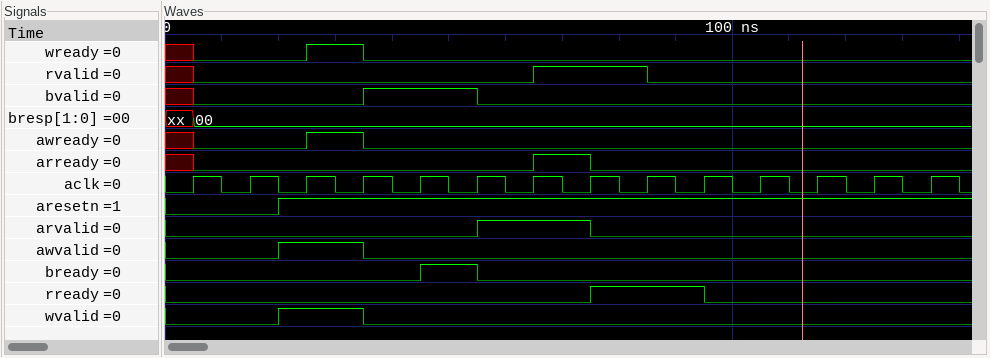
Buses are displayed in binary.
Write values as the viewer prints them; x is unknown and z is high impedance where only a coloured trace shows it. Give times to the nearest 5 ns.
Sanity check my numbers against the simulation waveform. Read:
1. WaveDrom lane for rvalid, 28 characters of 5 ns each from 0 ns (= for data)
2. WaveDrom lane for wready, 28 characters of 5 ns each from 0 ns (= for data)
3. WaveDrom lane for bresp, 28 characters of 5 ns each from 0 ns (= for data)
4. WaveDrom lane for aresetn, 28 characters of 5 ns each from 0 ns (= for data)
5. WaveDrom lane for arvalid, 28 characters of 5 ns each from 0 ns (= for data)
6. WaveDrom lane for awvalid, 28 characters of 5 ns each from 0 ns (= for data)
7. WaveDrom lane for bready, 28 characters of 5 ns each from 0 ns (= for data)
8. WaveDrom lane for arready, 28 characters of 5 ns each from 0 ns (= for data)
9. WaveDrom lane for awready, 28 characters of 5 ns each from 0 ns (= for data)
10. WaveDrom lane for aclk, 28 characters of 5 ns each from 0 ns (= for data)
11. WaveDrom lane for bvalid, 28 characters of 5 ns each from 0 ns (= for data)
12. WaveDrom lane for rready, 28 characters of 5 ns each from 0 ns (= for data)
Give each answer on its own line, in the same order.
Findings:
{name: 'rvalid', wave: 'x0...........1...0..........'}
{name: 'wready', wave: 'x0...1.0....................'}
{name: 'bresp', wave: 'x=..........................', data: '00'}
{name: 'aresetn', wave: '0...1.......................'}
{name: 'arvalid', wave: '0..........1...0............'}
{name: 'awvalid', wave: '0...1..0....................'}
{name: 'bready', wave: '0........1.0................'}
{name: 'arready', wave: 'x0...........1.0............'}
{name: 'awready', wave: 'x0...1.0....................'}
{name: 'aclk', wave: '0101010101010101010101010101'}
{name: 'bvalid', wave: 'x0.....1...0................'}
{name: 'rready', wave: '0..............1...0........'}
